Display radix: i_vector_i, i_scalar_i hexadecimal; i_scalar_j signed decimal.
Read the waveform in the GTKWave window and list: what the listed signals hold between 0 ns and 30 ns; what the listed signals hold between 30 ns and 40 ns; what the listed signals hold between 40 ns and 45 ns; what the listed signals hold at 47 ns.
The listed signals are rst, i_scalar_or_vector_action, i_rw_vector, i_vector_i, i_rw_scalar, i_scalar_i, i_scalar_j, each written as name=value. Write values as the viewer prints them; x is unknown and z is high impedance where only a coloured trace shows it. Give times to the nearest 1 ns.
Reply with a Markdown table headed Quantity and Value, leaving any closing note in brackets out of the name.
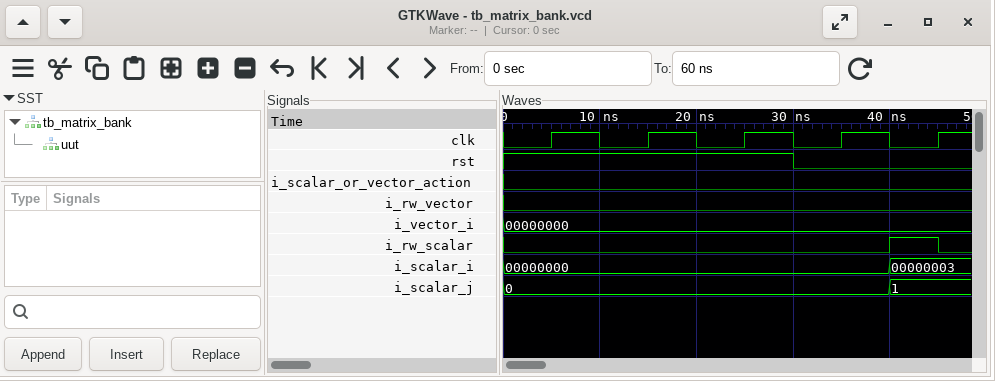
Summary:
| Quantity | Value |
|---|---|
| what the listed signals hold between 0 ns and 30 ns | rst=1, i_scalar_or_vector_action=0, i_rw_vector=0, i_vector_i=00000000, i_rw_scalar=0, i_scalar_i=00000000, i_scalar_j=0 |
| what the listed signals hold between 30 ns and 40 ns | rst=0, i_scalar_or_vector_action=0, i_rw_vector=0, i_vector_i=00000000, i_rw_scalar=0, i_scalar_i=00000000, i_scalar_j=0 |
| what the listed signals hold between 40 ns and 45 ns | rst=0, i_scalar_or_vector_action=0, i_rw_vector=0, i_vector_i=00000000, i_rw_scalar=1, i_scalar_i=00000003, i_scalar_j=1 |
| what the listed signals hold at 47 ns | rst=0, i_scalar_or_vector_action=0, i_rw_vector=0, i_vector_i=00000000, i_rw_scalar=0, i_scalar_i=00000003, i_scalar_j=1 |
